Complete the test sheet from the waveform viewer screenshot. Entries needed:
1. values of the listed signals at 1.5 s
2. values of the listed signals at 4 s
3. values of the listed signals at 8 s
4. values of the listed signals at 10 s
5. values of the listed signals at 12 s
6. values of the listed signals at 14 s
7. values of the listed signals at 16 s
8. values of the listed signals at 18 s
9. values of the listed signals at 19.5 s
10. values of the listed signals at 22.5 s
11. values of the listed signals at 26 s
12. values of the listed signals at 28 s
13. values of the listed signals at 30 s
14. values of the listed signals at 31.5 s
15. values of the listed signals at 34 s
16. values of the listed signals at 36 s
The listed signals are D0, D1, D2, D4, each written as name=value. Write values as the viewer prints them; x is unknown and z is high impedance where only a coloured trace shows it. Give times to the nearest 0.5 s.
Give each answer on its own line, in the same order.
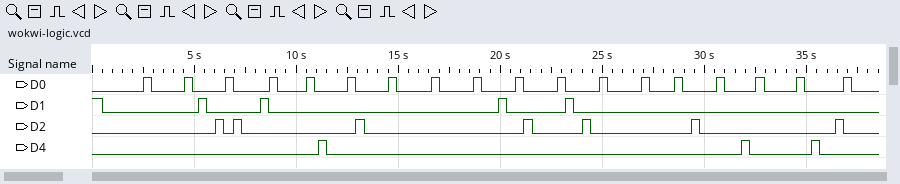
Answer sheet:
D0=0, D1=0, D2=0, D4=0
D0=0, D1=0, D2=0, D4=0
D0=0, D1=0, D2=0, D4=0
D0=0, D1=0, D2=0, D4=0
D0=0, D1=0, D2=0, D4=0
D0=0, D1=0, D2=0, D4=0
D0=0, D1=0, D2=0, D4=0
D0=0, D1=0, D2=0, D4=0
D0=0, D1=0, D2=0, D4=0
D0=0, D1=0, D2=0, D4=0
D0=0, D1=0, D2=0, D4=0
D0=0, D1=0, D2=0, D4=0
D0=0, D1=0, D2=0, D4=0
D0=0, D1=0, D2=0, D4=0
D0=0, D1=0, D2=0, D4=0
D0=0, D1=0, D2=0, D4=0
